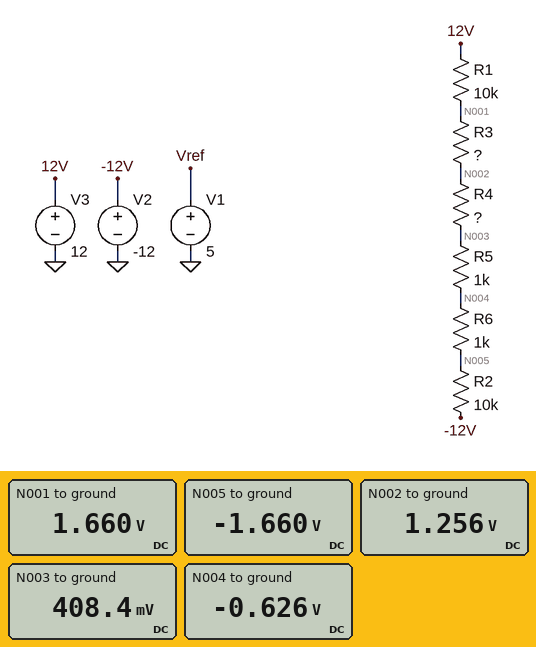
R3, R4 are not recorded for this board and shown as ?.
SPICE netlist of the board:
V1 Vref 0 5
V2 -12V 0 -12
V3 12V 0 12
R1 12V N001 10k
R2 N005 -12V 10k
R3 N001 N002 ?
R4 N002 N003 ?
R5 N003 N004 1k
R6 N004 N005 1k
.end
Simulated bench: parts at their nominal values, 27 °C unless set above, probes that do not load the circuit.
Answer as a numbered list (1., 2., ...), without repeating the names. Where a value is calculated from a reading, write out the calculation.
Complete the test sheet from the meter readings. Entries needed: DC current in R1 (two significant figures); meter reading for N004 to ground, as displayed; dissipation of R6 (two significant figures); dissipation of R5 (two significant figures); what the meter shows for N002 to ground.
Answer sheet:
1. (12 V - 1.66 V) / 10 kΩ = 1.0 mA
2. -0.626 V
3. (-626 mV - (-1.66 V))^2 / 1 kΩ = 1.1 mW
4. (408.4 mV - (-626 mV))^2 / 1 kΩ = 1.1 mW
5. 1.256 V
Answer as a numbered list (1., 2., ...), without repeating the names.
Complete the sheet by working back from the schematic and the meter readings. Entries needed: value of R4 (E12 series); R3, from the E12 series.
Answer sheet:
1. 820 Ω
2. 390 Ω
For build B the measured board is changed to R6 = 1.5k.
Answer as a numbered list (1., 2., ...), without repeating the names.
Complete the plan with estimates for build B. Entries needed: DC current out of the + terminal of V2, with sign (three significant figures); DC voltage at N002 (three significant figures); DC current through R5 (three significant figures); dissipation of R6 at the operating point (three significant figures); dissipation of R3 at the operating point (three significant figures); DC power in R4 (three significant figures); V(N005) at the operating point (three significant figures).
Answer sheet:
1. -1.01 mA
2. 1.48 V
3. 1.01 mA
4. 1.54 mW
5. 400 µW
6. 840 µW
7. -1.88 V
